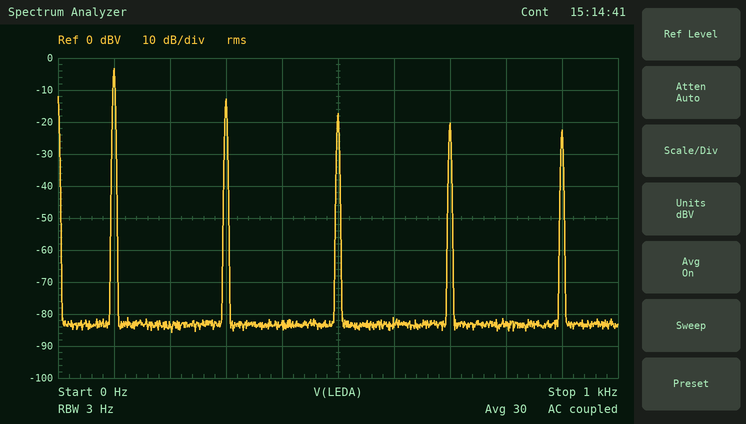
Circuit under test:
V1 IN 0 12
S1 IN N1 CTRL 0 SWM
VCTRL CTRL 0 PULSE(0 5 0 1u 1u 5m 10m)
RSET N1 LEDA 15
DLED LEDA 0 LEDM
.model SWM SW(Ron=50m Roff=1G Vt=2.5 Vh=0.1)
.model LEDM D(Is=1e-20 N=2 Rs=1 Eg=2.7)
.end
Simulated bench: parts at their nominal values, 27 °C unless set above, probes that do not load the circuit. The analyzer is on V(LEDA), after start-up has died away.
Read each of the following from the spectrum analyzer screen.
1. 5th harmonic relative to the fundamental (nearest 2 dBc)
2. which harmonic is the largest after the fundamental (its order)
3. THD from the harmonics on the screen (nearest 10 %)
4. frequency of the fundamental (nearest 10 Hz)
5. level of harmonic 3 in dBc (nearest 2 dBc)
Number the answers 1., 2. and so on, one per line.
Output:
1. -14 dBc
2. 3
3. 40 %
4. 100 Hz
5. -10 dBc
